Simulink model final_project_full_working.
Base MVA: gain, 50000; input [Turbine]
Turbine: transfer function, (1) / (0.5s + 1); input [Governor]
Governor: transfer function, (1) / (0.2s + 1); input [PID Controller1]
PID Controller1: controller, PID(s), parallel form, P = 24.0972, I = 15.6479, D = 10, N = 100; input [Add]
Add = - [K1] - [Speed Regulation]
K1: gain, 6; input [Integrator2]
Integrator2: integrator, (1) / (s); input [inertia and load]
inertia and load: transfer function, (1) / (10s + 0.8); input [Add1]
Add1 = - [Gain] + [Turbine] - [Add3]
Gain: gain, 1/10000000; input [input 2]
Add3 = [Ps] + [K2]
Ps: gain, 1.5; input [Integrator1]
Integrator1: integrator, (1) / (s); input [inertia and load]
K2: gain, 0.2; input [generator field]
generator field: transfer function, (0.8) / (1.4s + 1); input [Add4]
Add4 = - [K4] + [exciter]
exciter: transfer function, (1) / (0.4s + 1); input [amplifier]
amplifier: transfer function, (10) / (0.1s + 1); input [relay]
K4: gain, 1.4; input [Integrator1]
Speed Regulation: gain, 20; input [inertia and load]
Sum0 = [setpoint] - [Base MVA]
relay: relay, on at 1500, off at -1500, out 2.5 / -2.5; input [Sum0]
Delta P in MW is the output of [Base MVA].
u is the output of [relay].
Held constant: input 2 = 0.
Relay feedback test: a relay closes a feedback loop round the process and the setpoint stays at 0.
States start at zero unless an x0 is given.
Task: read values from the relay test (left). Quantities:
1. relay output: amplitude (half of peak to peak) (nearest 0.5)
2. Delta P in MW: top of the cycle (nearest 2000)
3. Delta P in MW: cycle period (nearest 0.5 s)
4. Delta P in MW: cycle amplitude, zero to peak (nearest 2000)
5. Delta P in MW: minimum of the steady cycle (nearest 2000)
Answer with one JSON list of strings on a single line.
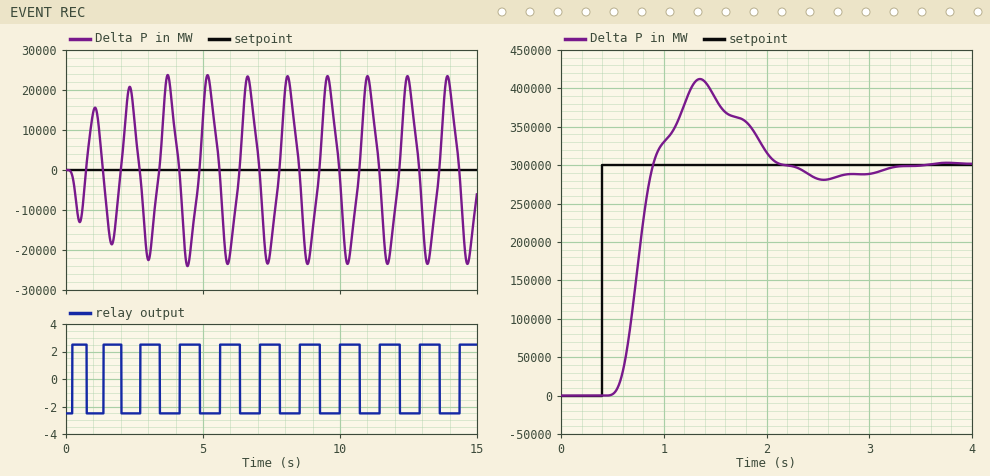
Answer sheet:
["2.5", "24000", "1.5 s", "24000", "-24000"]
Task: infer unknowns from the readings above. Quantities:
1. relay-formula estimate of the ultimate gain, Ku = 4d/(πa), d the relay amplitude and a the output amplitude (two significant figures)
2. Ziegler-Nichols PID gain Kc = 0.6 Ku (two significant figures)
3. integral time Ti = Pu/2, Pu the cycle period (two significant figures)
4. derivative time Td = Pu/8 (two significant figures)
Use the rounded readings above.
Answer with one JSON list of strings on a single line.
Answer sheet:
["0.00013", "0.000078", "0.75 s", "0.19 s"]
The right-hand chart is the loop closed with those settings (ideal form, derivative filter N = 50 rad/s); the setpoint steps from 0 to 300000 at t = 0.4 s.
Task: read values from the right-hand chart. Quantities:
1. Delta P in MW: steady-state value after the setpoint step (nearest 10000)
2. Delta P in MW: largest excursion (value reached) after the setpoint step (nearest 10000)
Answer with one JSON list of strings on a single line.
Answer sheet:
["300000", "410000"]
